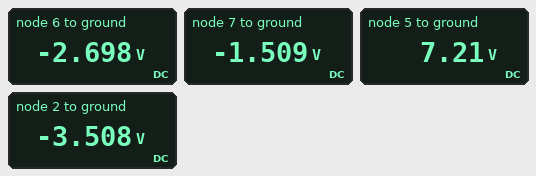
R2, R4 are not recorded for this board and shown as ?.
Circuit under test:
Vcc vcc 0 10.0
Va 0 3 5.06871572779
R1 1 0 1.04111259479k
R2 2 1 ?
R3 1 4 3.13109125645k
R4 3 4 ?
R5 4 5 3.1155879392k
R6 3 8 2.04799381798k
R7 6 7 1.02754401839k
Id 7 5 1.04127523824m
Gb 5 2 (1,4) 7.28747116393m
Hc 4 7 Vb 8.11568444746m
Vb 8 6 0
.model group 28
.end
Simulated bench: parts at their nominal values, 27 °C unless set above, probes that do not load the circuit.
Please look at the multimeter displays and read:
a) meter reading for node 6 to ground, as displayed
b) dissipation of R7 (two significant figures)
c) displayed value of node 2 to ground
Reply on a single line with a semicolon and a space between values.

-2.698 V; 1.4 mW; -3.508 V
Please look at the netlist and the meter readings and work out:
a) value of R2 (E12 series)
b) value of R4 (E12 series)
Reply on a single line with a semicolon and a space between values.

1 kΩ; 6.8 kΩ
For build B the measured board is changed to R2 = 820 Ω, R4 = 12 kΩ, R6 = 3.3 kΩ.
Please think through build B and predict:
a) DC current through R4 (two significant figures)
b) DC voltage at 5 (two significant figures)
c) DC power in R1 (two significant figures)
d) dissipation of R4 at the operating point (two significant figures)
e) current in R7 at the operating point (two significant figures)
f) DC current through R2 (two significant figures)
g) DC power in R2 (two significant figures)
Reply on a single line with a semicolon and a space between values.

330 µA; 6.2 V; 1.6 mW; 1.3 mW; 910 µA; 1.3 mA; 1.4 mW
